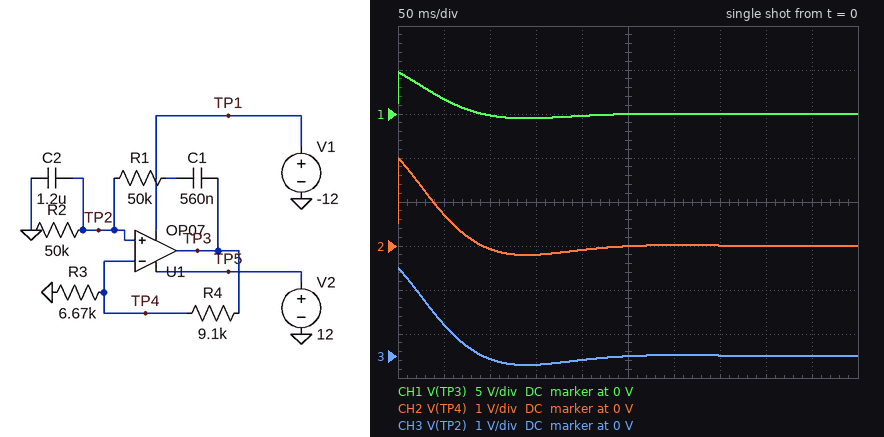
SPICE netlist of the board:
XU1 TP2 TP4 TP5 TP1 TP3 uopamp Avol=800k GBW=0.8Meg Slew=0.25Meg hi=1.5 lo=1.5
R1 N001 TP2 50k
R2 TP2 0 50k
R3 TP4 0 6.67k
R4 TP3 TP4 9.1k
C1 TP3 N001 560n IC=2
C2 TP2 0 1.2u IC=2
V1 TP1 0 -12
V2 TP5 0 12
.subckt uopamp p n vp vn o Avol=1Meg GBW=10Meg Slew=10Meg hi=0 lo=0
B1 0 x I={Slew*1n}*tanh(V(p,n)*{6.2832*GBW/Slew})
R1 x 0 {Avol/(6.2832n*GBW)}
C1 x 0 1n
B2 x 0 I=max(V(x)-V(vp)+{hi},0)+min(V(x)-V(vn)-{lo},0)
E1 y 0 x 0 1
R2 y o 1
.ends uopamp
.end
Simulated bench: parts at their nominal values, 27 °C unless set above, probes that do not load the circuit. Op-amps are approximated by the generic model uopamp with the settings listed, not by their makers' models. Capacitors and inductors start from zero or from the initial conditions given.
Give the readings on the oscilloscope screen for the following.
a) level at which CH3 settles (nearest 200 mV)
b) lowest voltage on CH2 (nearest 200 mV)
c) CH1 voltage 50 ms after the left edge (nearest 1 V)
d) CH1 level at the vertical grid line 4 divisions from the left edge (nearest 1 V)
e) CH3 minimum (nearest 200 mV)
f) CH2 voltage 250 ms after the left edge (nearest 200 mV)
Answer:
0 V
-200 mV
2 V
0 V
-200 mV
0 V
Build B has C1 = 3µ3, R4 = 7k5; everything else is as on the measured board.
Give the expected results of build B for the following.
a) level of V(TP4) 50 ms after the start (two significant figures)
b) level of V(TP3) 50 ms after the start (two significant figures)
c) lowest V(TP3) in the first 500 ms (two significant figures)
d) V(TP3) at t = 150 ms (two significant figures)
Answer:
500 mV
1.1 V
-4.5 V
-3.7 V
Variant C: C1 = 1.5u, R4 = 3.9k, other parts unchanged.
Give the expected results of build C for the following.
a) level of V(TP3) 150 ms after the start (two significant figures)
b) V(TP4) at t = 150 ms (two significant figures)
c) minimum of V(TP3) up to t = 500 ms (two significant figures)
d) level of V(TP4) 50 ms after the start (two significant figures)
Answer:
-900 mV
-570 mV
-910 mV
260 mV
